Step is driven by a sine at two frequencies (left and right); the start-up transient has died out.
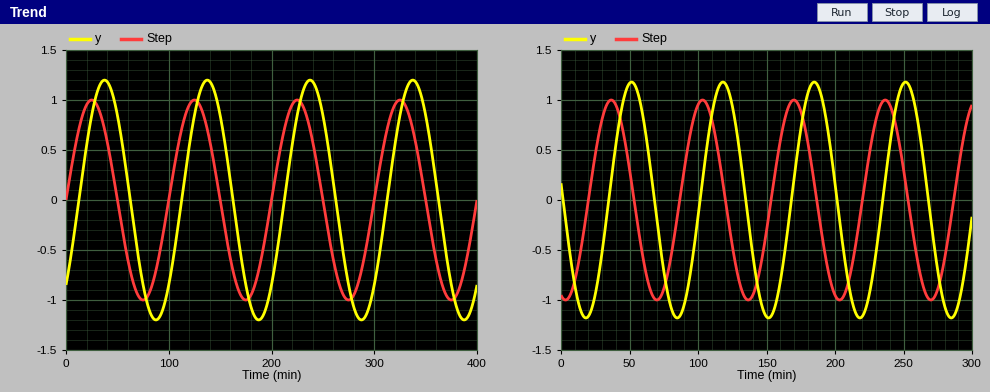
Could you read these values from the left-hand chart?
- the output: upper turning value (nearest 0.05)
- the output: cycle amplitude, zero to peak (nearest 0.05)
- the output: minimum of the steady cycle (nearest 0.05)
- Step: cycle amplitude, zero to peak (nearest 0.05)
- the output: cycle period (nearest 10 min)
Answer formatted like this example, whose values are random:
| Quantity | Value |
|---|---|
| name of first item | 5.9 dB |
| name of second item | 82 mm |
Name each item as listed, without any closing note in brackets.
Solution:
| Quantity | Value |
|---|---|
| the output: upper turning value | 1.20 |
| the output: cycle amplitude, zero to peak | 1.20 |
| the output: minimum of the steady cycle | -1.20 |
| Step: cycle amplitude, zero to peak | 1.00 |
| the output: cycle period | 100 min |
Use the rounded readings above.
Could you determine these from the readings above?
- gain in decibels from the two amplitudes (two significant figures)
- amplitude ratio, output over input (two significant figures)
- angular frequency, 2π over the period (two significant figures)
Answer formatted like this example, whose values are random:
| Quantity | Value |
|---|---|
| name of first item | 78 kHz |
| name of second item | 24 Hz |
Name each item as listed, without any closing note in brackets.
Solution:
| Quantity | Value |
|---|---|
| gain in decibels from the two amplitudes | 1.6 dB |
| amplitude ratio, output over input | 1.2 |
| angular frequency, 2π over the period | 0.063 rad/min |
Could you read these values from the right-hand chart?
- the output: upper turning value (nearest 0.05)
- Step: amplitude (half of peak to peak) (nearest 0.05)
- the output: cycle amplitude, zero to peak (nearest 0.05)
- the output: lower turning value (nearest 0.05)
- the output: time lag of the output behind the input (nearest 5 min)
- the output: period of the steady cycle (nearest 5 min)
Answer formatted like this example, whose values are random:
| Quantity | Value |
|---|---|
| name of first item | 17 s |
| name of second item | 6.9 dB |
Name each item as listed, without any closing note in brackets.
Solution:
| Quantity | Value |
|---|---|
| the output: upper turning value | 1.20 |
| Step: amplitude (half of peak to peak) | 1.00 |
| the output: cycle amplitude, zero to peak | 1.20 |
| the output: lower turning value | -1.20 |
| the output: time lag of the output behind the input | 15 min |
| the output: period of the steady cycle | 65 min |
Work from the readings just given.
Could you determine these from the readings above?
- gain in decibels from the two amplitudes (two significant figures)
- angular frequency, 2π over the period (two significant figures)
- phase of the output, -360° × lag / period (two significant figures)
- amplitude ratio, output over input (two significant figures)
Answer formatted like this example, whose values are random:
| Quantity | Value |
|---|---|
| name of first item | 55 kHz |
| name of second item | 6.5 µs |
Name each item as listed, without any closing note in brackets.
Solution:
| Quantity | Value |
|---|---|
| gain in decibels from the two amplitudes | 1.6 dB |
| angular frequency, 2π over the period | 0.097 rad/min |
| phase of the output, -360° × lag / period | -83° |
| amplitude ratio, output over input | 1.2 |
